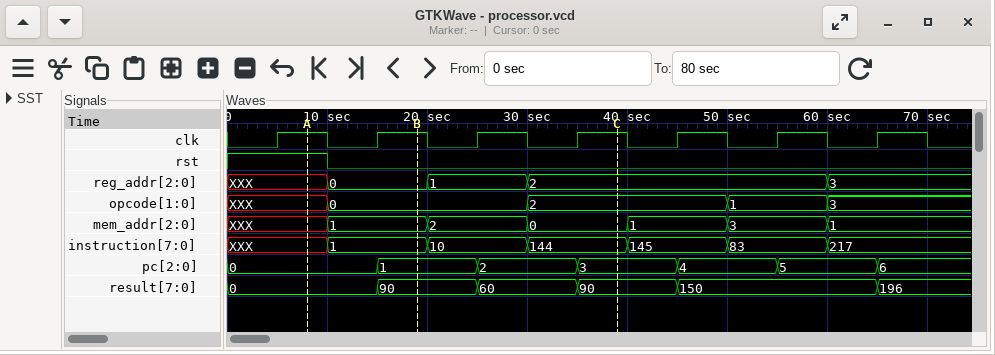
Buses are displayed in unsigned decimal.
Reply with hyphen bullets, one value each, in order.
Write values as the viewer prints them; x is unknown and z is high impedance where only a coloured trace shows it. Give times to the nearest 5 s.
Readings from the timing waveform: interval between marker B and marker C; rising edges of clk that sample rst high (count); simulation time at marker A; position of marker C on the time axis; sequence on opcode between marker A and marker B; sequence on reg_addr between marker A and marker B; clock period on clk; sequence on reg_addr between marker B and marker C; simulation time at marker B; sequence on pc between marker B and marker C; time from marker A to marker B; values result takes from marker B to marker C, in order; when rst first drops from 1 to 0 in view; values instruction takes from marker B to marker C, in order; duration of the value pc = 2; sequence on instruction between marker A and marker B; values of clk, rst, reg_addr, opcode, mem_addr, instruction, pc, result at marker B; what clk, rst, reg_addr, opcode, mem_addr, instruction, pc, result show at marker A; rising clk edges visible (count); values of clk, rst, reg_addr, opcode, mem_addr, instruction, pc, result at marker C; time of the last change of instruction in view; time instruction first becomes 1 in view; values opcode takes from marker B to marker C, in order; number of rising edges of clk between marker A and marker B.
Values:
- 20 s
- 1
- 10 s
- 40 s
- XXX, 0
- XXX, 0
- 10 s
- 0, 1, 2
- 20 s
- 1, 2, 3
- 10 s
- 90, 60, 90
- 10 s
- 1, 10, 144
- 10 s
- XXX, 1
- clk=1, rst=0, reg_addr=0, opcode=0, mem_addr=1, instruction=1, pc=1, result=90
- clk=1, rst=1, reg_addr=XXX, opcode=XXX, mem_addr=XXX, instruction=XXX, pc=0, result=0
- 7
- clk=1, rst=0, reg_addr=2, opcode=2, mem_addr=0, instruction=144, pc=3, result=90
- 60 s
- 10 s
- 0, 2
- 1
